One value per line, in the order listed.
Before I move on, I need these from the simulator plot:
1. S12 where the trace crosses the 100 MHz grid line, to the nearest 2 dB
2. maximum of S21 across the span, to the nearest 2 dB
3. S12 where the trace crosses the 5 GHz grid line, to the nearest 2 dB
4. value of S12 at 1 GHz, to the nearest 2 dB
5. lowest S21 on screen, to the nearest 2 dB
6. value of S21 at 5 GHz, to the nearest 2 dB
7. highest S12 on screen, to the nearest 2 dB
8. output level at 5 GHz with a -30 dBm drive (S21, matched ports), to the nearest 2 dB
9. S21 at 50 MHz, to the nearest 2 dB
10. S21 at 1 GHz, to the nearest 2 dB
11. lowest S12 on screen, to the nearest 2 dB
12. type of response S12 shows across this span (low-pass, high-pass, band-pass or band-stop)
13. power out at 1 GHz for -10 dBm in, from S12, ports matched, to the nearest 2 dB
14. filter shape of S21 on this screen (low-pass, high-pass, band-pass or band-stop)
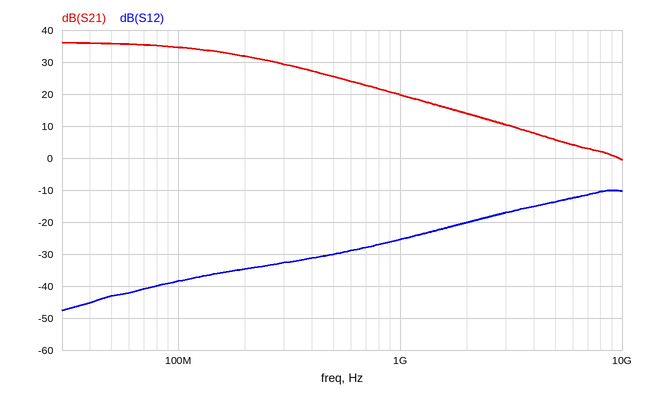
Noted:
-38 dB
36 dB
-14 dB
-26 dB
0 dB
6 dB
-10 dB
-24 dBm
36 dB
20 dB
-48 dB
high-pass
-36 dBm
low-pass
